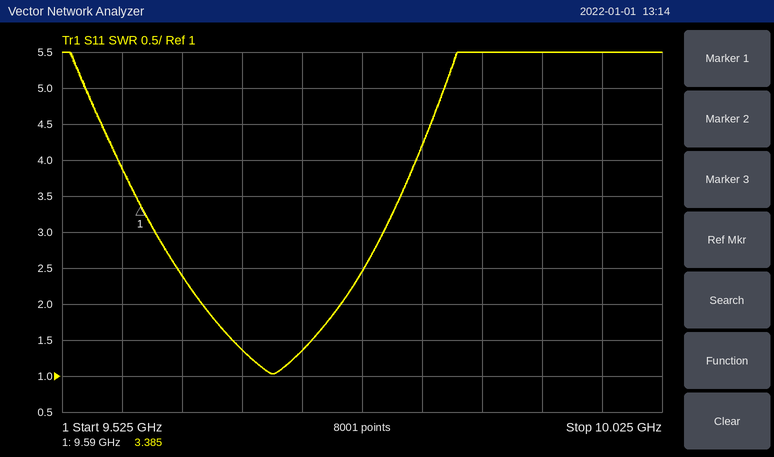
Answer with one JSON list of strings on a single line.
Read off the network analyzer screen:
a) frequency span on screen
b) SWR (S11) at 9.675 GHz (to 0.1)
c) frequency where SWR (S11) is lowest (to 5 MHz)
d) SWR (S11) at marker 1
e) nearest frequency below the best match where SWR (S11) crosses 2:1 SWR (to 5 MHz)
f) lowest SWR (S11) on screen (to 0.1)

["500 MHz", "1.4", "9.700 GHz", "3.385", "9.640 GHz", "1.0"]
